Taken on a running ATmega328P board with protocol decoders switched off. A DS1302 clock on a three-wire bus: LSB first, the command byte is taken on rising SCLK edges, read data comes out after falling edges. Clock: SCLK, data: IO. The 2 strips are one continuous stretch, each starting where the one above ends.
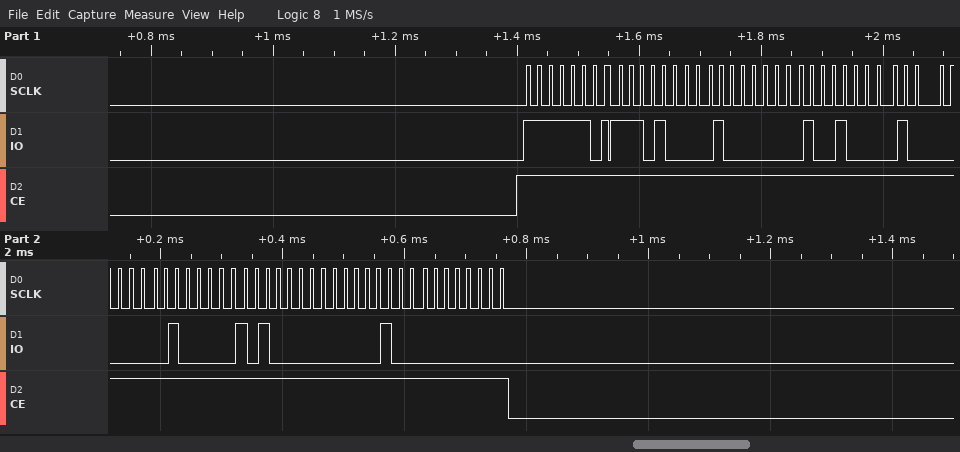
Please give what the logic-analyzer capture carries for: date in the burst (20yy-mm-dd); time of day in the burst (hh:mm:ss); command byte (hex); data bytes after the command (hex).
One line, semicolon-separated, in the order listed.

2020-04-02; 12:02:17; 0xBF; 17 02 12 02 04 05 20 00
